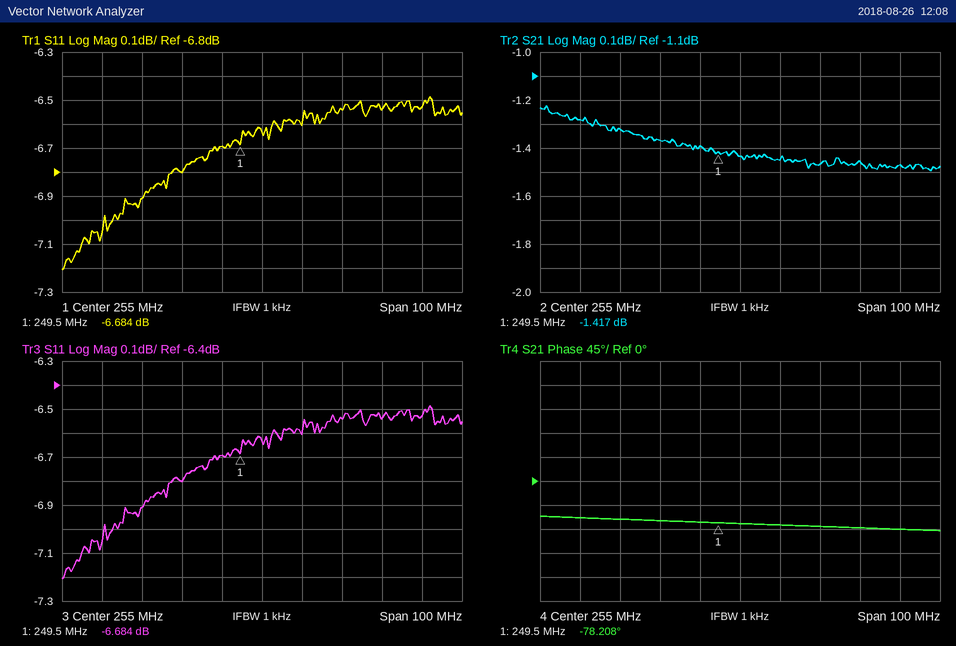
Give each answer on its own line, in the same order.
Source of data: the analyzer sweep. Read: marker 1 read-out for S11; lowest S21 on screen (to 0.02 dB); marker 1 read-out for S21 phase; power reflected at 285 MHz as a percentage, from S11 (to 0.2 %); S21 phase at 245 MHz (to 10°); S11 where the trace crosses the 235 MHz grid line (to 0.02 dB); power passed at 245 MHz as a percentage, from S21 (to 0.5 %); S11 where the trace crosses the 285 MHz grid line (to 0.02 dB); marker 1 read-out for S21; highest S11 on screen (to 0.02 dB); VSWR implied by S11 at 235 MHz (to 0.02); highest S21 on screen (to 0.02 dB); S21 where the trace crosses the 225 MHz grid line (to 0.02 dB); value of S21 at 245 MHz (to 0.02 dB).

-6.684 dB
-1.50 dB
-78.208°
22.2 %
-80°
-6.80 dB
72.5 %
-6.54 dB
-1.417 dB
-6.48 dB
2.68
-1.22 dB
-1.32 dB
-1.40 dB
